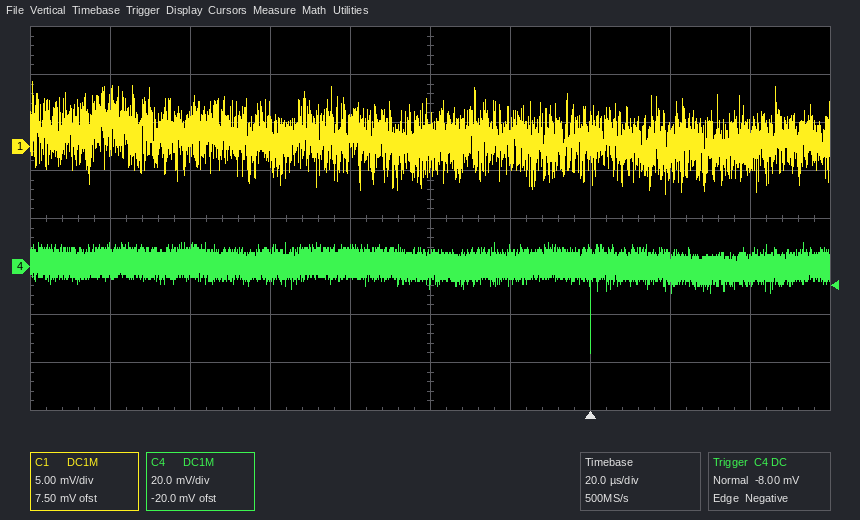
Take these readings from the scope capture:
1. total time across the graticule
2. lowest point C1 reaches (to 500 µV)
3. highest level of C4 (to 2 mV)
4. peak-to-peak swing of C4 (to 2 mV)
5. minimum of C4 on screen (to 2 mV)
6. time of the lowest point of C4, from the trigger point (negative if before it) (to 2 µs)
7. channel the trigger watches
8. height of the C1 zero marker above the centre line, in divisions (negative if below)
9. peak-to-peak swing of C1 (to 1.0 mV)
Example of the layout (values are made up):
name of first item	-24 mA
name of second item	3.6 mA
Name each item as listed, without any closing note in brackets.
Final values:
total time across the graticule	200 µs
lowest point C1 reaches	-5.0 mV
highest level of C4	10 mV
peak-to-peak swing of C4	46 mV
minimum of C4 on screen	-36 mV
time of the lowest point of C4, from the trigger point (negative if before it)	0 µs
channel the trigger watches	C4
height of the C1 zero marker above the centre line, in divisions	+1.5 div
peak-to-peak swing of C1	12.0 mV
